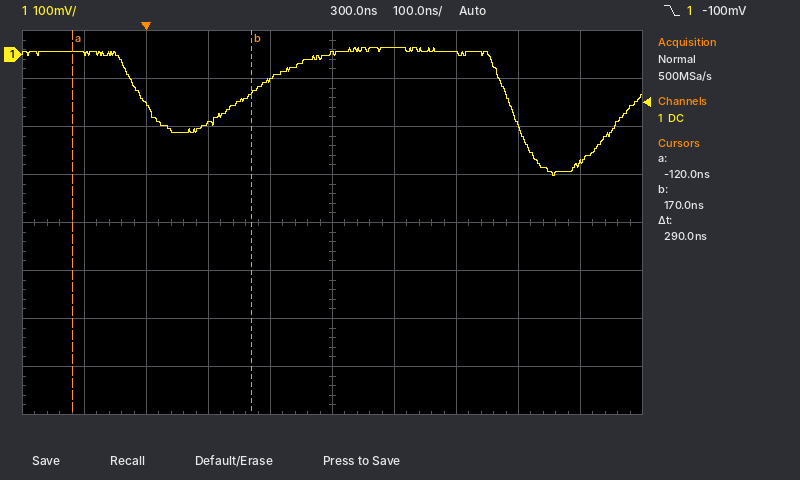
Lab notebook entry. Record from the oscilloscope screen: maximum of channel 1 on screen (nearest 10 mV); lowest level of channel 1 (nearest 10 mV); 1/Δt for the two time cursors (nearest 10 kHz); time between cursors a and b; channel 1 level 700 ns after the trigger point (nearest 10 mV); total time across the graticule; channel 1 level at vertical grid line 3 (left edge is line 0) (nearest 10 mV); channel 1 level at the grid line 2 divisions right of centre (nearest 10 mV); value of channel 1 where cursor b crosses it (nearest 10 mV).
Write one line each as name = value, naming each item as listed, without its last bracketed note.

maximum of channel 1 on screen = 10 mV
lowest level of channel 1 = -250 mV
1/Δt for the two time cursors = 3.45 MHz
time between cursors a and b = 290 ns
channel 1 level 700 ns after the trigger point = -230 mV
total time across the graticule = 1 µs
channel 1 level at vertical grid line 3 (left edge is line 0) = -140 mV
channel 1 level at the grid line 2 divisions right of centre = 0 mV
value of channel 1 where cursor b crosses it = -80 mV
